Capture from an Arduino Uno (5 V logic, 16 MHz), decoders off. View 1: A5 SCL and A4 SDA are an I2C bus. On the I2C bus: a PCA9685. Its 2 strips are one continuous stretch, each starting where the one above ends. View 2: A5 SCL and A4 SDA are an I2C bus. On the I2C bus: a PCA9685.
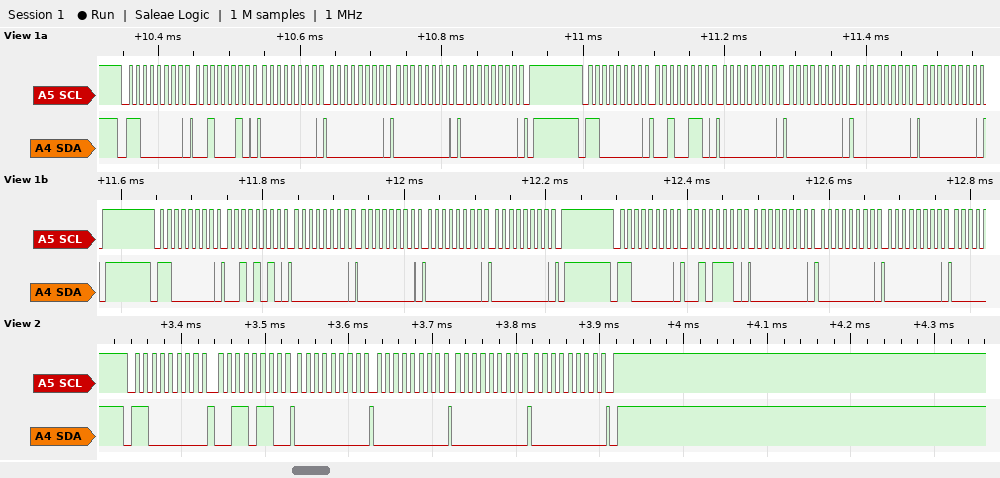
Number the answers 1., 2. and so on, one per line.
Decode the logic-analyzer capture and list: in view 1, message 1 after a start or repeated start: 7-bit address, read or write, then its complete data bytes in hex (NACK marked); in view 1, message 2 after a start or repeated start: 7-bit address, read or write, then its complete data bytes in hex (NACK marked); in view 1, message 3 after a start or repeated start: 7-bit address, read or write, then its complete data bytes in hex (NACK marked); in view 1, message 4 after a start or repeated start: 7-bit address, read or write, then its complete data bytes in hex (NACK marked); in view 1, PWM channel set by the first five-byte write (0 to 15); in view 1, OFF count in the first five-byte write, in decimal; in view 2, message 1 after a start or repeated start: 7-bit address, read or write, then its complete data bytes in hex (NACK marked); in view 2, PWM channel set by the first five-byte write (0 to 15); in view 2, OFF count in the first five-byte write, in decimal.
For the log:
1. 0x60 write: 22 00 00 00 00
2. 0x60 write: 26 00 00 00 00
3. 0x60 write: 2A 00 00 00 00
4. 0x60 write: 2E 00 00 00
5. 7
6. 0
7. 0x60 write: 36 00 00 00 00
8. 12
9. 0
